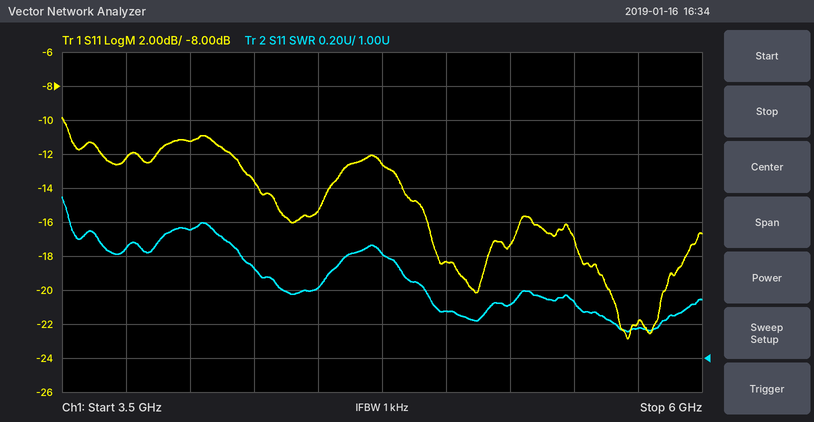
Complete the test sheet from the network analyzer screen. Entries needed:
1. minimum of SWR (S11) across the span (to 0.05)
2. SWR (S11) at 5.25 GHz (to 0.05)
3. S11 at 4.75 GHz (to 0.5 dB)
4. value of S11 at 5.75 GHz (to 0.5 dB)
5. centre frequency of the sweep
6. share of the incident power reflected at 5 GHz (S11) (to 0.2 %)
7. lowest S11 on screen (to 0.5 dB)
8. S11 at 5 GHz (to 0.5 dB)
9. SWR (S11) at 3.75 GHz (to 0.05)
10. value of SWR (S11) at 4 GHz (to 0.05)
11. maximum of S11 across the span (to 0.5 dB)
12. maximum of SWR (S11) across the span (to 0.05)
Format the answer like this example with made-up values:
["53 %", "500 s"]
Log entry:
["1.15", "1.30", "-12.5 dB", "-22.0 dB", "4.75 GHz", "1.4 %", "-23.0 dB", "-18.5 dB", "1.65", "1.75", "-10.0 dB", "1.95"]
